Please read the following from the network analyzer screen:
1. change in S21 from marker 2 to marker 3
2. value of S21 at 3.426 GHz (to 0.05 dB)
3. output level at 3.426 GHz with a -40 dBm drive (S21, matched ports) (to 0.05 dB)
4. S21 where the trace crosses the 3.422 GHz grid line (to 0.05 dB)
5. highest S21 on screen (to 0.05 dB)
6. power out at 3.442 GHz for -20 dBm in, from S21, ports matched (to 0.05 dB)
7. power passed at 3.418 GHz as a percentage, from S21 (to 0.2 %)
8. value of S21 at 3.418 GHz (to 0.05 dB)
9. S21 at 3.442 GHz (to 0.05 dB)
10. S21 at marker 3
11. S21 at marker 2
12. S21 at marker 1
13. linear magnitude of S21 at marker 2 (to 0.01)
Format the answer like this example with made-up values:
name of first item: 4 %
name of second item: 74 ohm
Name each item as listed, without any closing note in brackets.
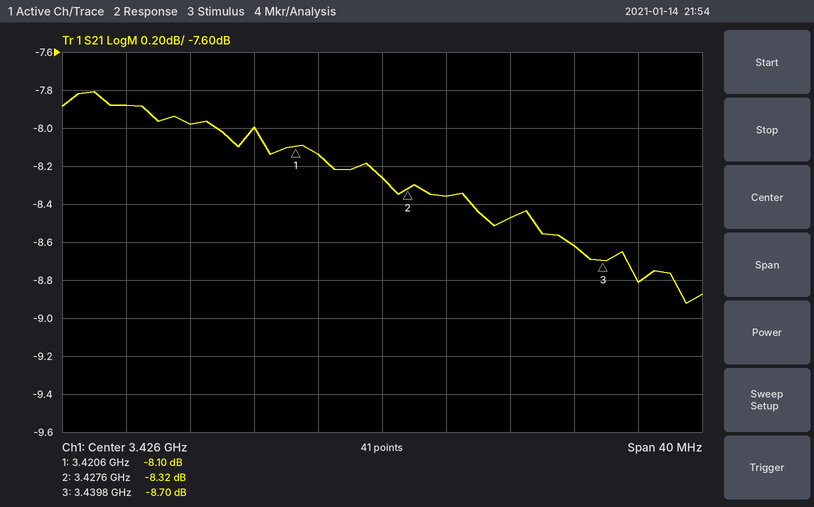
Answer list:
change in S21 from marker 2 to marker 3: -0.38 dB
value of S21 at 3.426 GHz: -8.25 dB
output level at 3.426 GHz with a -40 dBm drive (S21, matched ports): -48.25 dBm
S21 where the trace crosses the 3.422 GHz grid line: -8.15 dB
highest S21 on screen: -7.80 dB
power out at 3.442 GHz for -20 dBm in, from S21, ports matched: -28.80 dBm
power passed at 3.418 GHz as a percentage, from S21: 15.8 %
value of S21 at 3.418 GHz: -8.00 dB
S21 at 3.442 GHz: -8.80 dB
S21 at marker 3: -8.70 dB
S21 at marker 2: -8.32 dB
S21 at marker 1: -8.10 dB
linear magnitude of S21 at marker 2: 0.38
